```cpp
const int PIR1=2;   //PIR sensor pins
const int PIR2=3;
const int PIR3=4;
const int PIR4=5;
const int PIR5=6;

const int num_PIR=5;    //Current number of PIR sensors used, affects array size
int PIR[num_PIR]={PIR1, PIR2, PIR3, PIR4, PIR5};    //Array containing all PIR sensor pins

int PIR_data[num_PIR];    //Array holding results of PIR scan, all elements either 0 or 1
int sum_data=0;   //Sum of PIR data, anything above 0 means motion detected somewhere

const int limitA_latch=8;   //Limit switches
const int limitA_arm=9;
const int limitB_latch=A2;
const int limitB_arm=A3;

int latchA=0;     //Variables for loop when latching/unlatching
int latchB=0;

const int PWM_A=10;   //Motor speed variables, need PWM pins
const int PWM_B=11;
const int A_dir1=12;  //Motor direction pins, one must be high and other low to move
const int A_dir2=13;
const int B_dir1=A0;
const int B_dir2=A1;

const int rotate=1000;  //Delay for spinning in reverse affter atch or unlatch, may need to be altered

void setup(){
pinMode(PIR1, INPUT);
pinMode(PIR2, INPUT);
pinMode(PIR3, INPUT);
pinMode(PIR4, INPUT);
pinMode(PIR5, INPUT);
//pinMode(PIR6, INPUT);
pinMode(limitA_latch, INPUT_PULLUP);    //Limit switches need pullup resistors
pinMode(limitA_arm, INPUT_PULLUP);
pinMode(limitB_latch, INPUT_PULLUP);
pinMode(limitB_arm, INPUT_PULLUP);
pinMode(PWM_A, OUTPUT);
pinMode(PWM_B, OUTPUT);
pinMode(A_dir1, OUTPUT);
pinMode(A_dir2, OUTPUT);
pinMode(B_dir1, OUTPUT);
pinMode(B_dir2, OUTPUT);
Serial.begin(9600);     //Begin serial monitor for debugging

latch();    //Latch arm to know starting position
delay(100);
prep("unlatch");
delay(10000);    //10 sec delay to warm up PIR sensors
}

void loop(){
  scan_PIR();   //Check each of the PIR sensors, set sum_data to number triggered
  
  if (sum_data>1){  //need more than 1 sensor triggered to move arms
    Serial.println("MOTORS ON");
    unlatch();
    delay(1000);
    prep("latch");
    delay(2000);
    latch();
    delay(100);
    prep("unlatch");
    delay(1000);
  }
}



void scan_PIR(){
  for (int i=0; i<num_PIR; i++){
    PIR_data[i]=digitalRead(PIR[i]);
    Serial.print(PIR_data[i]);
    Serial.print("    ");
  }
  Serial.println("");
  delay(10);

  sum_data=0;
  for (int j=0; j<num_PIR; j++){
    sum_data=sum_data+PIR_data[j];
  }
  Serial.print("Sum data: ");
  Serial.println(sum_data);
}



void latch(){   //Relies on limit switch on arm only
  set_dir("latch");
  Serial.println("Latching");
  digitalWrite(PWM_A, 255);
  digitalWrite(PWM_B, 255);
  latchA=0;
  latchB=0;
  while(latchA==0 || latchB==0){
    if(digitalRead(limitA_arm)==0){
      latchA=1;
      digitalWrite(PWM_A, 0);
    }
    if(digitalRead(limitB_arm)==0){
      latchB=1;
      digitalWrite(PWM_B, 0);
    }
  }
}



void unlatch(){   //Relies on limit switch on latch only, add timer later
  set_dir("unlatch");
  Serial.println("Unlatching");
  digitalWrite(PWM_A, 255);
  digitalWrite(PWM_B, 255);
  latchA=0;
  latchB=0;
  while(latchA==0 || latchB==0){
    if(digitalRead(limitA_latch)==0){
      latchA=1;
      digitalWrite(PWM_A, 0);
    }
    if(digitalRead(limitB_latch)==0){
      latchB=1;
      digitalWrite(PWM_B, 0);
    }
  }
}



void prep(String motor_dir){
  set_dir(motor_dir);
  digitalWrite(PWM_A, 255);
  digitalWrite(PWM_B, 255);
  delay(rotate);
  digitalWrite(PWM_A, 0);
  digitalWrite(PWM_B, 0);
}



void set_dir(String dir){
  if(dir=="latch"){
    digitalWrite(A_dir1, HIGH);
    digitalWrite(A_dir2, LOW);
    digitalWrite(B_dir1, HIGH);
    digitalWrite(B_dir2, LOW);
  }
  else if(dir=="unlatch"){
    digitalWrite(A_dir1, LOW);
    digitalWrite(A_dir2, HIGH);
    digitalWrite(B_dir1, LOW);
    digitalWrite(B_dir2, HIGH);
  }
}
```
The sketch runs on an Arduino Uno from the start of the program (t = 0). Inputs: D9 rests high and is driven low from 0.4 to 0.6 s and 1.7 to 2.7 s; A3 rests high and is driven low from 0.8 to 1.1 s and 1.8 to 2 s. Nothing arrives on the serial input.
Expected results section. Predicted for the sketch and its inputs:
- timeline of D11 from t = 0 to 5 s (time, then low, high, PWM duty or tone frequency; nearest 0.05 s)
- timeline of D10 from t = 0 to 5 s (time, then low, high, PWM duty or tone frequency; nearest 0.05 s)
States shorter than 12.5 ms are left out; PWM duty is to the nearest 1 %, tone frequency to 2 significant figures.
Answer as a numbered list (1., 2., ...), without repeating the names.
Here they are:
1. 0 s high; 0.8 s low; 0.9 s high; 1.9 s low
2. 0 s high; 0.4 s low; 0.9 s high; 1.9 s low
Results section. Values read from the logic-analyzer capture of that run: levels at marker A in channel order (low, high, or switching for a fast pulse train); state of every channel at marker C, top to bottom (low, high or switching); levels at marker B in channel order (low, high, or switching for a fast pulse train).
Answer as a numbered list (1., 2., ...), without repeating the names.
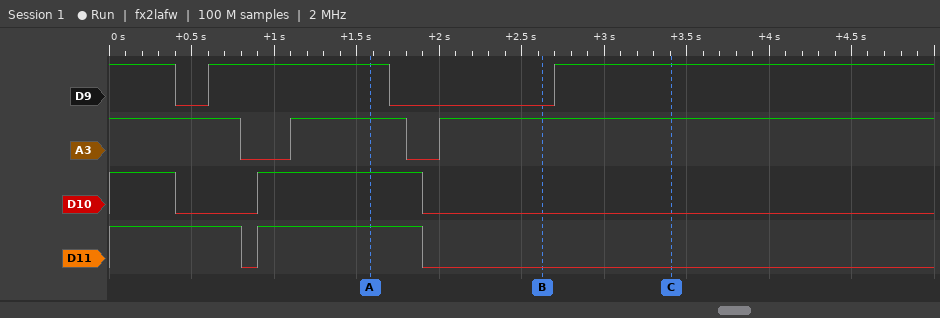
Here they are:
1. D9 high, A3 high, D10 high, D11 high
2. D9 high, A3 high, D10 low, D11 low
3. D9 low, A3 high, D10 low, D11 low
